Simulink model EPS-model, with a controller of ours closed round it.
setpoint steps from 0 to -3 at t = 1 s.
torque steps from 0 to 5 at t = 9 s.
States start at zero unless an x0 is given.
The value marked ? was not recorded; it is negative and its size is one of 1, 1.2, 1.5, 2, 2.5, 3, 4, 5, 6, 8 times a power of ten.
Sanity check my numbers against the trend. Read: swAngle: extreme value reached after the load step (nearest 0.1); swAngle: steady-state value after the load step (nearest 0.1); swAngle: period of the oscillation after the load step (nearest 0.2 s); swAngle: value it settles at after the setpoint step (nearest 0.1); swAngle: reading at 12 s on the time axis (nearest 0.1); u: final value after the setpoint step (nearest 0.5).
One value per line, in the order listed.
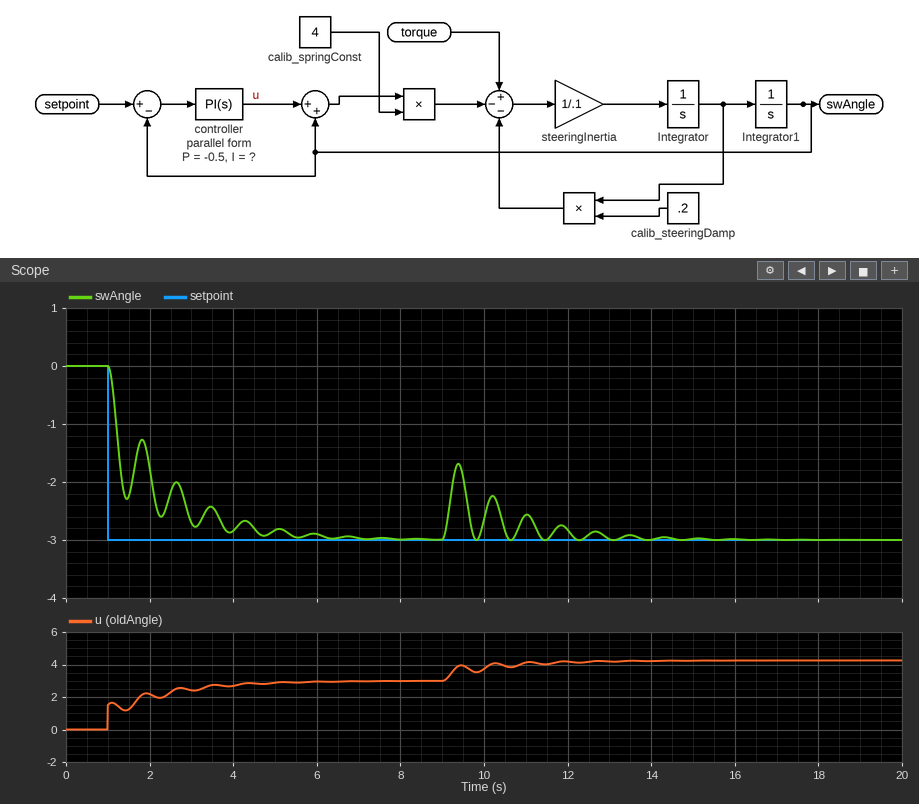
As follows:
-1.7
-3.0
0.8 s
-3.0
-2.8
3.0
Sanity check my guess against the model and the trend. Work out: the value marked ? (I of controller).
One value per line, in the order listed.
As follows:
-1
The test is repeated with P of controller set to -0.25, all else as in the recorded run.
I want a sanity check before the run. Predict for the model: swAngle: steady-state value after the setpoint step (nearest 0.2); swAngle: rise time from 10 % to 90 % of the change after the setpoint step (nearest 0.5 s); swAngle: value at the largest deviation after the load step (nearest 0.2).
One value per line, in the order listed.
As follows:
-3.0
2.0 s
-1.4
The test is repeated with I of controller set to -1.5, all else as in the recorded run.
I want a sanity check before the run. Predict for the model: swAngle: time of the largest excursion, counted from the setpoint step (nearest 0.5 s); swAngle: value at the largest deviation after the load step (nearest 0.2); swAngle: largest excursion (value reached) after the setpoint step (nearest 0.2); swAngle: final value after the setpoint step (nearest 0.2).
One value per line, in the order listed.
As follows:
3.0 s
-1.8
-3.2
-3.0
